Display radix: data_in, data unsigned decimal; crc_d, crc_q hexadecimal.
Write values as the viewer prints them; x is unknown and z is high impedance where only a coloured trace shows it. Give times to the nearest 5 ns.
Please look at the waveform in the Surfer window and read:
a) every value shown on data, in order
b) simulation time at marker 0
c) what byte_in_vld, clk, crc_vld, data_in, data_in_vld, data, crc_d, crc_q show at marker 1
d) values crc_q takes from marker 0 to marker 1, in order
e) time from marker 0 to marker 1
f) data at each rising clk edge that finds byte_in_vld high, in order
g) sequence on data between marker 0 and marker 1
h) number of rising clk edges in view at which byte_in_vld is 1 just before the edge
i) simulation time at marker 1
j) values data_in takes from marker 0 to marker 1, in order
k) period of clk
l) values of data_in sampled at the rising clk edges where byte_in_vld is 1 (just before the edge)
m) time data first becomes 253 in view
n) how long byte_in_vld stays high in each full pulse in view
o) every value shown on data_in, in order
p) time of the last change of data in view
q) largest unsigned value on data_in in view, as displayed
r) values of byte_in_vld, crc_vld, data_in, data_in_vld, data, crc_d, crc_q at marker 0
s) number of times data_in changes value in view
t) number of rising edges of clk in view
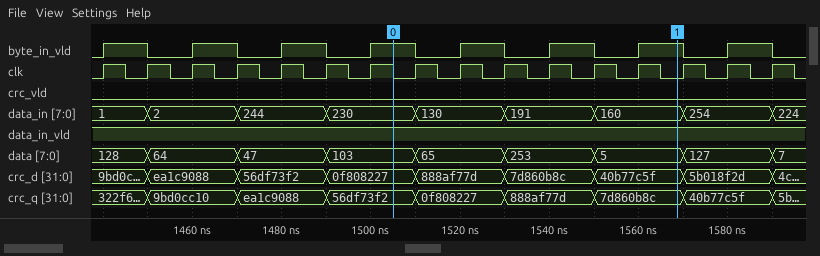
128, 64, 47, 103, 65, 253, 5, 127, 7
1505 ns
byte_in_vld=1, clk=0, crc_vld=0, data_in=160, data_in_vld=1, data=5, crc_d=40b77c5f, crc_q=7d860b8c
56df73f2, 0f808227, 888af77d, 7d860b8c
65 ns
128, 64, 47, 103, 65, 253, 5, 127
103, 65, 253, 5
8
1570 ns
230, 130, 191, 160
10 ns
1, 2, 244, 230, 130, 191, 160, 254
1530 ns
10 ns, 10 ns, 10 ns, 10 ns, 10 ns, 10 ns, 10 ns, 10 ns
1, 2, 244, 230, 130, 191, 160, 254, 224
1590 ns
254
byte_in_vld=1, crc_vld=0, data_in=230, data_in_vld=1, data=103, crc_d=0f808227, crc_q=56df73f2
8
16
